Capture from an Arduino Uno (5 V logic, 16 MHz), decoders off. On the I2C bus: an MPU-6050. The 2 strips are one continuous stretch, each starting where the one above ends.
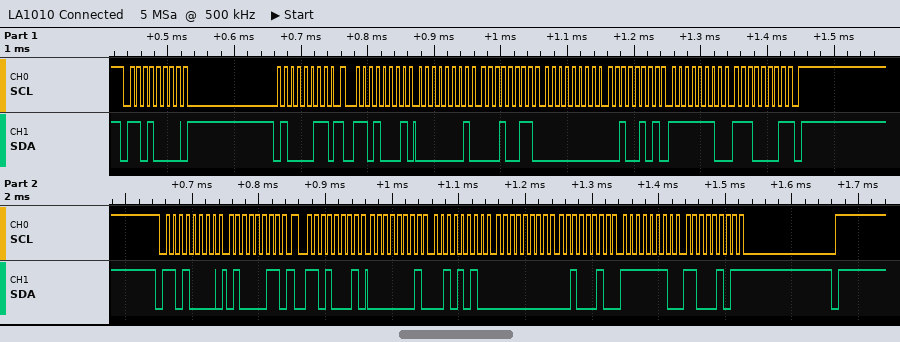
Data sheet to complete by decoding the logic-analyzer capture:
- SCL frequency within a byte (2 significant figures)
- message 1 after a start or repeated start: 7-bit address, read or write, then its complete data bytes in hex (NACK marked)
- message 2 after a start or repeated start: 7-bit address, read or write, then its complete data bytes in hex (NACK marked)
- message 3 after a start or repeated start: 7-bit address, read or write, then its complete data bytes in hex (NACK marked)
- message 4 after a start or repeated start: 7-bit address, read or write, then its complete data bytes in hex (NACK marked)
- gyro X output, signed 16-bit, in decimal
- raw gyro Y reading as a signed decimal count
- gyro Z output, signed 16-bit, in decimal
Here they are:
100 kHz
0x68 write: 43
0x68 read: 01 13 00 25 FE E1 NACK
0x68 write: 43
0x68 read: 01 2A 00 22 FE C5 NACK
275
37
-287
